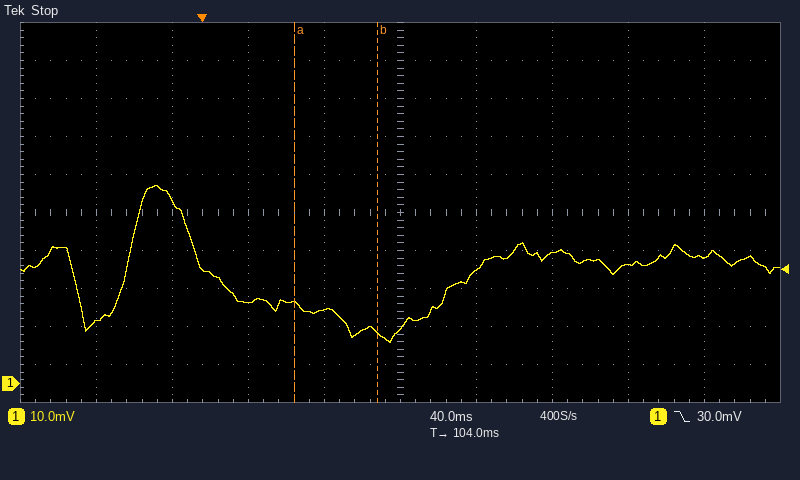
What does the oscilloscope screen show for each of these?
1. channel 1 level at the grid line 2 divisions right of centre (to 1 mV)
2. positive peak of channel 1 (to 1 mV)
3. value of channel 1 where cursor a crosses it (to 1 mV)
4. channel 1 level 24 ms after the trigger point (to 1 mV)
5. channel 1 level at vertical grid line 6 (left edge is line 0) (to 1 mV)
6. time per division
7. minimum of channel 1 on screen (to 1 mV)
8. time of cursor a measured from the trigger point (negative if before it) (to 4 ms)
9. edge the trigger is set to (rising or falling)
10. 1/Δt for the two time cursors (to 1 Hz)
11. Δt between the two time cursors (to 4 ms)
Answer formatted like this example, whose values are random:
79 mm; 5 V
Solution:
34 mV; 52 mV; 21 mV; 21 mV; 30 mV; 40 ms; 11 mV; +48 ms; falling; 23 Hz; 44 ms
